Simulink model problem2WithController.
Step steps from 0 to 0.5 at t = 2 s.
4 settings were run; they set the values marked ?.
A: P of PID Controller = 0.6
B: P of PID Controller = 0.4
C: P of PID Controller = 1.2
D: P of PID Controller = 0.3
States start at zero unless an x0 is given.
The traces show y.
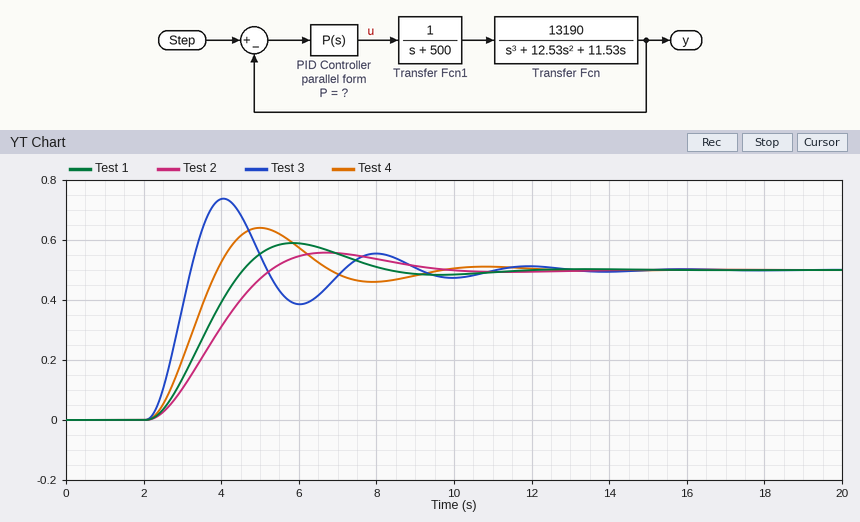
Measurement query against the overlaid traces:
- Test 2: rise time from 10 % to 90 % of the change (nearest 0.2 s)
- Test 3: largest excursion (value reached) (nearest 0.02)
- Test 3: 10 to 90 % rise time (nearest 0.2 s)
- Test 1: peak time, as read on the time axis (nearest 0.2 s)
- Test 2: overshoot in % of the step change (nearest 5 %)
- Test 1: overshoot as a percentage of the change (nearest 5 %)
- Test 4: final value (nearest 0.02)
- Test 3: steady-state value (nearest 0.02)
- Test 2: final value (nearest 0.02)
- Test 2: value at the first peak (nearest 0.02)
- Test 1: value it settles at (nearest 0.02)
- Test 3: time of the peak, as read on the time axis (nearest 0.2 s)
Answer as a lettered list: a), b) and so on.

a) 2.2 s
b) 0.74
c) 0.8 s
d) 5.8 s
e) 10 %
f) 20 %
g) 0.50
h) 0.50
i) 0.50
j) 0.56
k) 0.50
l) 4.0 s
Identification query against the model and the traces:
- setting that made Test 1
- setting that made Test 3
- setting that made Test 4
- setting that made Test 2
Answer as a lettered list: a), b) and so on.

a) B
b) C
c) A
d) D
